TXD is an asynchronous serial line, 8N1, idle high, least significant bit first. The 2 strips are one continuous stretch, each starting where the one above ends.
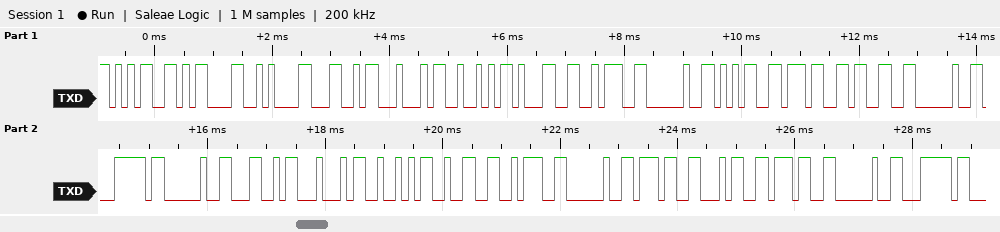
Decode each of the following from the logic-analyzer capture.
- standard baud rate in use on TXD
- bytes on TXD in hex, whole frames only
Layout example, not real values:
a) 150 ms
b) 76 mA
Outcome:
a) 9600 baud
b) 35 0D 0A 4C 44 52 31 3A 20 35 37 33 20 7C 20 4C 44 52 32 3A 20 37 34 37 20 7C
